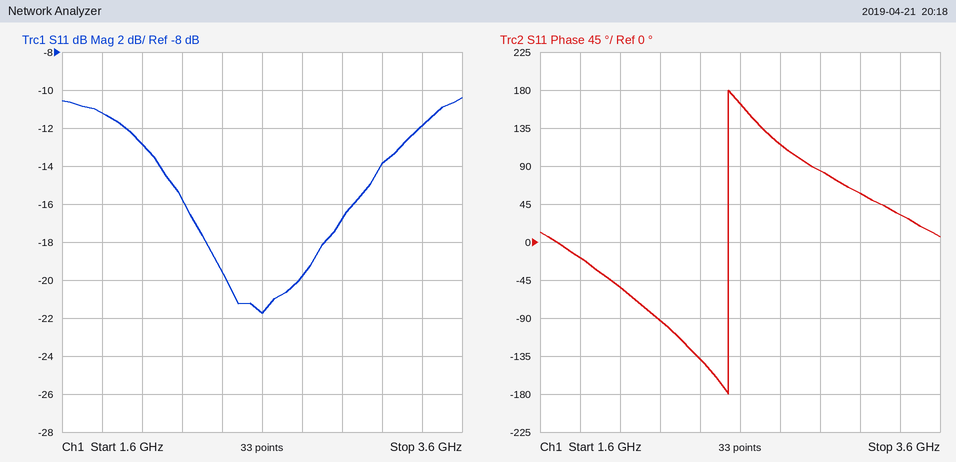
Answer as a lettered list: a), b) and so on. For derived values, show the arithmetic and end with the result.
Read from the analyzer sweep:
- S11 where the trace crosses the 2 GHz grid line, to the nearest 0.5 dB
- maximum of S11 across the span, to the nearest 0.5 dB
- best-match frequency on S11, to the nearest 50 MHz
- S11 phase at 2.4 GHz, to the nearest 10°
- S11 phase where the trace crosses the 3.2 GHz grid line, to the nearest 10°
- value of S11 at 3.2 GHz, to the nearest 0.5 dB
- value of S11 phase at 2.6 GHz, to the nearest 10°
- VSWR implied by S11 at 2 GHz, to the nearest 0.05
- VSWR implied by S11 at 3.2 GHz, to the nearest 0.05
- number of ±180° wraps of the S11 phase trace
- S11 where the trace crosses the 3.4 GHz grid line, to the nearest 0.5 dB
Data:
a) -13.0 dB
b) -10.5 dB
c) 2.60 GHz
d) -140°
e) 60°
f) -14.0 dB
g) 160°
h) |Γ| = 10^(-13/20) = 0.2239; VSWR = (1 + 0.2239)/(1 − 0.2239) ≈ 1.58, so 1.60 to the nearest 0.05
i) |Γ| = 10^(-14/20) = 0.1995; VSWR = (1 + 0.1995)/(1 − 0.1995) ≈ 1.50
j) 1
k) -12.0 dB
